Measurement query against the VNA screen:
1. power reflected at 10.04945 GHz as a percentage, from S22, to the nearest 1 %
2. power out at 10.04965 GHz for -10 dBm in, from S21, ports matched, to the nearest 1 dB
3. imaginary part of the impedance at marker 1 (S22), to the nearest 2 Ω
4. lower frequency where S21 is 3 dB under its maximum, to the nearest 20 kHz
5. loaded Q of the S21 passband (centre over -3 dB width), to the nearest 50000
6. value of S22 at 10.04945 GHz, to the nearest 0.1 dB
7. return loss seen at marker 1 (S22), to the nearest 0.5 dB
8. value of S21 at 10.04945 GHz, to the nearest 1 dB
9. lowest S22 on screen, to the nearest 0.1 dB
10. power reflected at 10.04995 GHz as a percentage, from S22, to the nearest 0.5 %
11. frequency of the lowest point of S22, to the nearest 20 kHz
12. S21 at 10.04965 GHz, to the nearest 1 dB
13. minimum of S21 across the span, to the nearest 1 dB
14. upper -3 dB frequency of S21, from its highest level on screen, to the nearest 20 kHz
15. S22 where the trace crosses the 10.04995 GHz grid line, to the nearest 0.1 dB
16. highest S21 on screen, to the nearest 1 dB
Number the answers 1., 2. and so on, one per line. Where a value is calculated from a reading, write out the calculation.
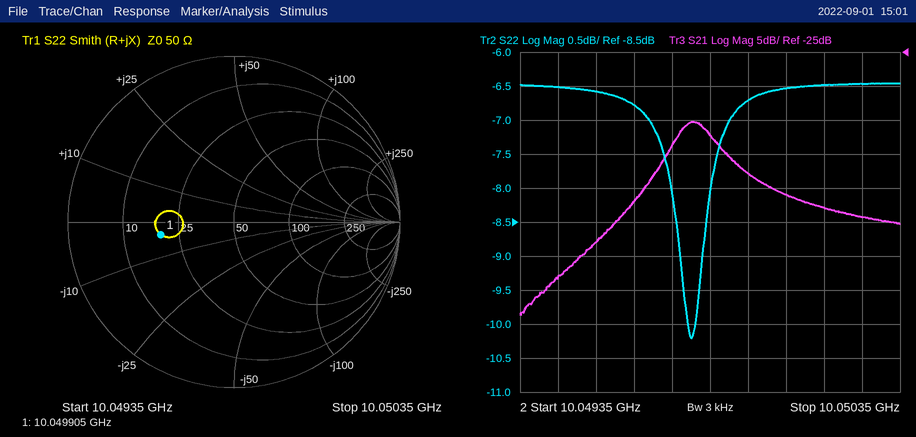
1. 10^(-6.5/10) ≈ 22 %
2. -10 dBm + (-47 dB) = -57 dBm
3. -4 Ω
4. 10.04976 GHz
5. 10.0498 GHz / 100 kHz ≈ 100498, so 100000 to the nearest 50000
6. -6.5 dB
7. 7.0 dB
8. -58 dB
9. -10.2 dB
10. 10^(-6.7/10) ≈ 21.4 %, so 21.5 % to the nearest 0.5 %
11. 10.04980 GHz
12. -47 dB
13. -64 dB
14. 10.04986 GHz
15. -6.7 dB
16. -35 dB
